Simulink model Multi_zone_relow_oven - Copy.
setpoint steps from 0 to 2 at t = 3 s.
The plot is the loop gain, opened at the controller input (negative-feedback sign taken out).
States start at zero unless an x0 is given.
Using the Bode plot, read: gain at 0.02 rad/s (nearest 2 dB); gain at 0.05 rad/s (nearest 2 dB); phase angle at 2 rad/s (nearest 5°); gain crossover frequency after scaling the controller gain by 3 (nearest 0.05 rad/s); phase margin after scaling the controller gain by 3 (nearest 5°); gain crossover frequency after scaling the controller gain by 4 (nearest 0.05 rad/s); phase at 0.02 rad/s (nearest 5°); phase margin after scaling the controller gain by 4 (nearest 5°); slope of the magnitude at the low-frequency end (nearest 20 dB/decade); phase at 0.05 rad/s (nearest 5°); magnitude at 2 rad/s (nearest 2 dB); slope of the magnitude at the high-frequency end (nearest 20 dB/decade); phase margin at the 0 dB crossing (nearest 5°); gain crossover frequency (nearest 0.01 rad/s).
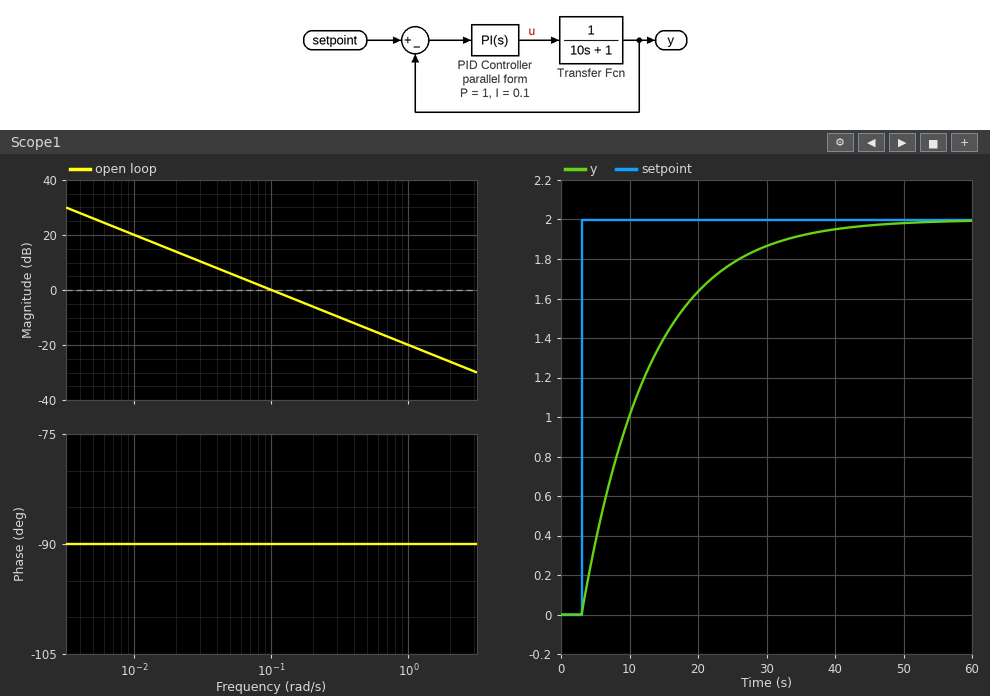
14 dB
6 dB
-90°
0.30 rad/s
90°
0.40 rad/s
-90°
90°
-20 dB/decade
-90°
-26 dB
-20 dB/decade
90°
0.10 rad/s
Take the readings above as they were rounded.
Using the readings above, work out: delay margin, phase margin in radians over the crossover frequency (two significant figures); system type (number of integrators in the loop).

16 s
1
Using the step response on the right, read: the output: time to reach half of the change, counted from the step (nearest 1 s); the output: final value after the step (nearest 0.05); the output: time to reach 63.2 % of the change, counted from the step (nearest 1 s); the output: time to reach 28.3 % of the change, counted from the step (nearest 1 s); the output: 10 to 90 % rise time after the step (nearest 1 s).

7 s
2.00
10 s
3 s
22 s
